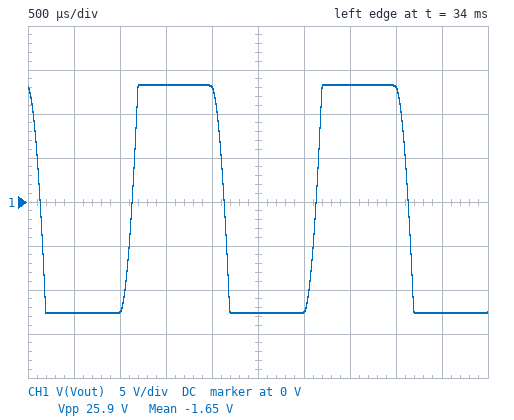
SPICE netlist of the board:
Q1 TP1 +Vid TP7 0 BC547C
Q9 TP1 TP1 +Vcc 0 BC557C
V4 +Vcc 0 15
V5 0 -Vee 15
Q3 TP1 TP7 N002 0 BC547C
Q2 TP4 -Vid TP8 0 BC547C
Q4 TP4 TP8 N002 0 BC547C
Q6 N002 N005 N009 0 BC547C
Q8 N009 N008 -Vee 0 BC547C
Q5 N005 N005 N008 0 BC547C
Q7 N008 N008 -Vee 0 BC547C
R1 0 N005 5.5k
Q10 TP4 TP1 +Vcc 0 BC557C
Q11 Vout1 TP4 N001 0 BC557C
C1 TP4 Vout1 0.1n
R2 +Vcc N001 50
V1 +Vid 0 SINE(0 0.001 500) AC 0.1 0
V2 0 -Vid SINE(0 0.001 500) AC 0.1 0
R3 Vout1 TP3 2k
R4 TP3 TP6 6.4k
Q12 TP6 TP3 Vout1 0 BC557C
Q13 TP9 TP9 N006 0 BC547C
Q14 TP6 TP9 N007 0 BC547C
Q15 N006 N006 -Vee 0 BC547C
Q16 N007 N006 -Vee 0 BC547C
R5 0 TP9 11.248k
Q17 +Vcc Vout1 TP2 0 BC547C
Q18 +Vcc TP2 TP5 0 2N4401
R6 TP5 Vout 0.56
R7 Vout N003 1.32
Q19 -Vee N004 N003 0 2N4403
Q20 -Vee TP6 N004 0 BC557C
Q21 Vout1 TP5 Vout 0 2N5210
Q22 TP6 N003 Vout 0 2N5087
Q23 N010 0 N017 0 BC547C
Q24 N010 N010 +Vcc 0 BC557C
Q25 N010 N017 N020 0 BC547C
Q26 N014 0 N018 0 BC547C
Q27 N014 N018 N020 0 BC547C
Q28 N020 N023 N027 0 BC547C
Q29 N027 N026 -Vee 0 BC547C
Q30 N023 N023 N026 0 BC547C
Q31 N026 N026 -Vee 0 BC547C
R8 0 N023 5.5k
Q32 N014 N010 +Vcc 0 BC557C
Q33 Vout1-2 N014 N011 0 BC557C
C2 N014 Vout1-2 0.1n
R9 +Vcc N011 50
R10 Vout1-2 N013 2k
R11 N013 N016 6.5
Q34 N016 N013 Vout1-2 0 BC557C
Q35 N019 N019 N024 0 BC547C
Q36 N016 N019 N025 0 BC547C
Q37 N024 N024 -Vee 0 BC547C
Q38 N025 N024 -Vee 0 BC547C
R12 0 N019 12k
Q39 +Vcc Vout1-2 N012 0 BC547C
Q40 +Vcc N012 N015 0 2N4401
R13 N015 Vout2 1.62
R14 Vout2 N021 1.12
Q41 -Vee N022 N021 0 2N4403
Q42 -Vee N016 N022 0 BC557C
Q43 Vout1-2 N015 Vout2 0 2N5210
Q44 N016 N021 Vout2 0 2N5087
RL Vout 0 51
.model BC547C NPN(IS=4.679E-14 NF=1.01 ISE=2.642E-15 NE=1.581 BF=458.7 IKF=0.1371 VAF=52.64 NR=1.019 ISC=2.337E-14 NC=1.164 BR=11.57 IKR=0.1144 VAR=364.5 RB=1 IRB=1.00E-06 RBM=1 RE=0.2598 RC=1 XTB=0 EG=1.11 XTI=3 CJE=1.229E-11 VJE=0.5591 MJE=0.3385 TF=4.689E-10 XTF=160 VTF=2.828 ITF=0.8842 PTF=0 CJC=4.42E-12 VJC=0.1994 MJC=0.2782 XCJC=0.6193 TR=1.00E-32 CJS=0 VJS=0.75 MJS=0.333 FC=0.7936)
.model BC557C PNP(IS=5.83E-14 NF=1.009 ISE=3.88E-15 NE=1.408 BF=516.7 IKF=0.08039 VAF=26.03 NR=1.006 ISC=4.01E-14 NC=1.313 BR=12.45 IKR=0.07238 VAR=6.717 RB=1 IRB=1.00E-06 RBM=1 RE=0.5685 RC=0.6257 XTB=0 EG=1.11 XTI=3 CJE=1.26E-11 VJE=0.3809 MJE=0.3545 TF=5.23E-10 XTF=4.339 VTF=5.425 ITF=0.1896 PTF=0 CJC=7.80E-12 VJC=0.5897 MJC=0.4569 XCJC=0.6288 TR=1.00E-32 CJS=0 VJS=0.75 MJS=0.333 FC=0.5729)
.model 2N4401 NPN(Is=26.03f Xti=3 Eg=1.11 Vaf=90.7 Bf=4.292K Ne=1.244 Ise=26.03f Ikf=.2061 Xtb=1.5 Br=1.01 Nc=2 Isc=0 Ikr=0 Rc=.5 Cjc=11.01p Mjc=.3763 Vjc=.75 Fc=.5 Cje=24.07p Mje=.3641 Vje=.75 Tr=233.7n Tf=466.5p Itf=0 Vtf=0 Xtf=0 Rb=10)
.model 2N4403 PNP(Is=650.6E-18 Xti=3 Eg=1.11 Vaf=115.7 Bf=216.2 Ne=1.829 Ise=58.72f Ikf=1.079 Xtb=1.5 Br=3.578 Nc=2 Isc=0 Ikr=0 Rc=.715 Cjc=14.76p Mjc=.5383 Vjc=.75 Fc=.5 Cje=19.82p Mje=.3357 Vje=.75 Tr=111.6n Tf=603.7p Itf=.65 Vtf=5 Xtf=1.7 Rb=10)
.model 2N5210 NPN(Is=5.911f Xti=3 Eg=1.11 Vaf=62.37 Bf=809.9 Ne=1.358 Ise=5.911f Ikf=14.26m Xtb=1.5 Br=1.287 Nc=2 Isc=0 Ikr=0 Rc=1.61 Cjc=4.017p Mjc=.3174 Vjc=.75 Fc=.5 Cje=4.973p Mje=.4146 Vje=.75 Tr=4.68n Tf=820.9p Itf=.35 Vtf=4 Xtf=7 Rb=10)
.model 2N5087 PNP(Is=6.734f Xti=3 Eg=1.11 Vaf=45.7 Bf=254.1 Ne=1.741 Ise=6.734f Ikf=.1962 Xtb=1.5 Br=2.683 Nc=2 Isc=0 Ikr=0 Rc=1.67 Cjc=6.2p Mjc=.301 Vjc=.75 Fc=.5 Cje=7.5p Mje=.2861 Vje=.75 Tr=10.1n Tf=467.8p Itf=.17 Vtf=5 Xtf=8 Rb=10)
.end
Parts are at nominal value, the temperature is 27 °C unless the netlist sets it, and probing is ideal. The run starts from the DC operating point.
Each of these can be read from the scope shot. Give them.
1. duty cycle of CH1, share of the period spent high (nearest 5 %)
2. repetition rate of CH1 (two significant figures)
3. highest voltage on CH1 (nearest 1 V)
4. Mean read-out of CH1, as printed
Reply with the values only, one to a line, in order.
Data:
50 %
500 Hz
13 V
-1.65 V
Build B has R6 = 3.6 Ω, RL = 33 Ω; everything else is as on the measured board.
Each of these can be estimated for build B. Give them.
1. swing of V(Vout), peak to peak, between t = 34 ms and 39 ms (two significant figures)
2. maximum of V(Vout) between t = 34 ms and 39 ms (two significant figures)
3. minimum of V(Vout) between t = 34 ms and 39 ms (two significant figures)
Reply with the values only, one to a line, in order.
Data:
19 V
6.9 V
-12 V
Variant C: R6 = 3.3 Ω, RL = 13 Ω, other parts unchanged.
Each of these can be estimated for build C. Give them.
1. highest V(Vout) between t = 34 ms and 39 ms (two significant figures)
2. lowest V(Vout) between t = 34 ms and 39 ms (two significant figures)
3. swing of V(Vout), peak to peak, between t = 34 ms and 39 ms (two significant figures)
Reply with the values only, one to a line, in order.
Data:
3.0 V
-6.6 V
9.5 V
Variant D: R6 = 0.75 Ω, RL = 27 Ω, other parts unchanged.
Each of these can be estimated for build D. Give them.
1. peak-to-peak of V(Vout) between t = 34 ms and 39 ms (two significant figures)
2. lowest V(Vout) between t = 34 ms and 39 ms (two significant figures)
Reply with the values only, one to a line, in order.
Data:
25 V
-12 V
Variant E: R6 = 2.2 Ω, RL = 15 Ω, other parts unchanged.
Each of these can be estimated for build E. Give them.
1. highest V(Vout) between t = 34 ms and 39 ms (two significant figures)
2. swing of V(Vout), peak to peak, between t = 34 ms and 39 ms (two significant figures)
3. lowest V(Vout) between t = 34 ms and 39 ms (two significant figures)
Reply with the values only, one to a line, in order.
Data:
5.1 V
13 V
-7.6 V
